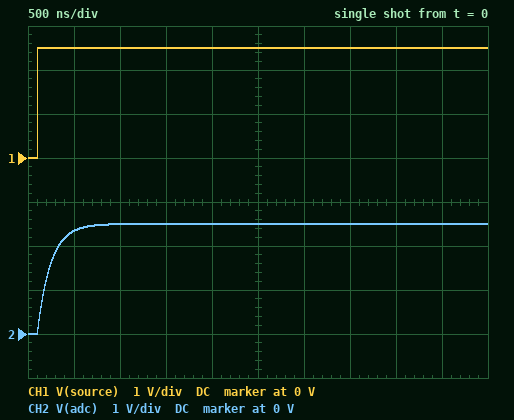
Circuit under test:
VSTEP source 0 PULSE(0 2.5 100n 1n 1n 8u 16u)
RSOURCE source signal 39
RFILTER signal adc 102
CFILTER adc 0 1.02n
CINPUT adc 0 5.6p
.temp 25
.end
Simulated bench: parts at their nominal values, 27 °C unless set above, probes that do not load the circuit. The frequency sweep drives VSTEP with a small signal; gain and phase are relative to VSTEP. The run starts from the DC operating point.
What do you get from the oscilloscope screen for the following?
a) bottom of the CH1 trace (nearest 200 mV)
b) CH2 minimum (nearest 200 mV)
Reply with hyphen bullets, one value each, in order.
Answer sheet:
- 0 V
- 0 V
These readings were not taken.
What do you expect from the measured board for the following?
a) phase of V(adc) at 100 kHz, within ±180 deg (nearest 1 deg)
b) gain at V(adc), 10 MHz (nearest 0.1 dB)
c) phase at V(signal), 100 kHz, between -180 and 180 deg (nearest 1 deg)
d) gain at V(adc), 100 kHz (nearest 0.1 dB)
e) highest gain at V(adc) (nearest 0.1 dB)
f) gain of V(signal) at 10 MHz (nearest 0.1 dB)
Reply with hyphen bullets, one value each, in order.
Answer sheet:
- -5 deg
- -19.2 dB
- -1 deg
- 0 dB
- 0 dB
- -2.8 dB
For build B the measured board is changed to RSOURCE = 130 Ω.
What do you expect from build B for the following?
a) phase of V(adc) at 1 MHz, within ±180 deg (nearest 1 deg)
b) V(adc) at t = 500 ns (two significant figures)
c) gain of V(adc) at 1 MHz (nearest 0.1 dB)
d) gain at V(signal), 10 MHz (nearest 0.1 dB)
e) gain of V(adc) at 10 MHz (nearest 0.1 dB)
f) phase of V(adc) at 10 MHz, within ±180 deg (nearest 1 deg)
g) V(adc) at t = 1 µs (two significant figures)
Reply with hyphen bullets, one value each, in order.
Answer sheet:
- -56 deg
- 2.0 V
- -5.1 dB
- -7.1 dB
- -23.5 dB
- -86 deg
- 2.4 V
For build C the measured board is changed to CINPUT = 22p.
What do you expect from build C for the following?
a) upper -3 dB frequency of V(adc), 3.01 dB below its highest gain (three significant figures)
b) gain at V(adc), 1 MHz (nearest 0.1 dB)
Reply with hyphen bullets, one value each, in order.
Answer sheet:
- 1.08 MHz
- -2.7 dB
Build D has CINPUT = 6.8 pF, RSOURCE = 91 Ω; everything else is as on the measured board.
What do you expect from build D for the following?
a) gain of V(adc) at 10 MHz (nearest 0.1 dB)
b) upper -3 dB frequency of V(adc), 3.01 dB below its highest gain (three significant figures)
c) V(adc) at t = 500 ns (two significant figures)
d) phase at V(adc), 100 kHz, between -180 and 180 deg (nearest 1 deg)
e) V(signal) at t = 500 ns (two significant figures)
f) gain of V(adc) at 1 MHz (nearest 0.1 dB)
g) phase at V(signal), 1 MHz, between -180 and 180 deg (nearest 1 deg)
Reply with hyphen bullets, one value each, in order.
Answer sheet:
- -21.9 dB
- 803 kHz
- 2.2 V
- -7 deg
- 2.3 V
- -4.1 dB
- -18 deg
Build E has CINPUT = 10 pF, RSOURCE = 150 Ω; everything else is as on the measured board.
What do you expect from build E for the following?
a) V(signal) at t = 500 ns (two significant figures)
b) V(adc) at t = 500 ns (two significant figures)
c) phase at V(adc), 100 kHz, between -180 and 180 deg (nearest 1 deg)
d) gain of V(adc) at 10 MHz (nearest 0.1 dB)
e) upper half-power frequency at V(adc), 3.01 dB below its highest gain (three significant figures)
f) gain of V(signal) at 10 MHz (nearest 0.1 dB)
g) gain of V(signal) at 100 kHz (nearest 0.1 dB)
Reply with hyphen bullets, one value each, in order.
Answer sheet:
- 2.2 V
- 2.0 V
- -9 deg
- -24.3 dB
- 613 kHz
- -7.8 dB
- -0.1 dB
